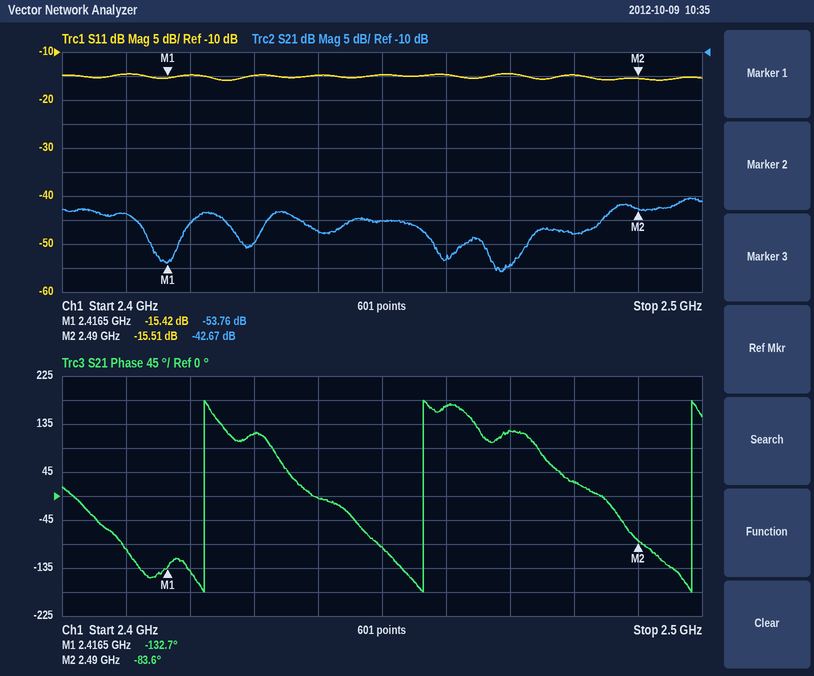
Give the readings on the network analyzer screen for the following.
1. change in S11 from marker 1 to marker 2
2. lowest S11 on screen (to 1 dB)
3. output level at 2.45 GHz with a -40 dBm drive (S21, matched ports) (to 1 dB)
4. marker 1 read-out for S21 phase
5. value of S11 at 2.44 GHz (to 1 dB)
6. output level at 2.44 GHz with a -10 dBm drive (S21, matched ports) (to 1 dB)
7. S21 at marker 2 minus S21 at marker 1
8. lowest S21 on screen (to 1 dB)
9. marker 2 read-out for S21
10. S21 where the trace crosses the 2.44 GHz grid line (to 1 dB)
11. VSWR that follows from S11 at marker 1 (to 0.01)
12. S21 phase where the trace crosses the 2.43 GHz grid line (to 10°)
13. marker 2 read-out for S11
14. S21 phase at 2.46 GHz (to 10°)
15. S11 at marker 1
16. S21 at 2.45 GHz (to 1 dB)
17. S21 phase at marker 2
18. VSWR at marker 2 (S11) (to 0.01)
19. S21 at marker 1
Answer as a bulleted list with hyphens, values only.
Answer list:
- -0.09 dB
- -16 dB
- -85 dBm
- -132.7°
- -15 dB
- -57 dBm
- 11.09 dB
- -56 dB
- -42.67 dB
- -47 dB
- 1.41
- 120°
- -15.51 dB
- 170°
- -15.42 dB
- -45 dB
- -83.6°
- 1.40
- -53.76 dB
